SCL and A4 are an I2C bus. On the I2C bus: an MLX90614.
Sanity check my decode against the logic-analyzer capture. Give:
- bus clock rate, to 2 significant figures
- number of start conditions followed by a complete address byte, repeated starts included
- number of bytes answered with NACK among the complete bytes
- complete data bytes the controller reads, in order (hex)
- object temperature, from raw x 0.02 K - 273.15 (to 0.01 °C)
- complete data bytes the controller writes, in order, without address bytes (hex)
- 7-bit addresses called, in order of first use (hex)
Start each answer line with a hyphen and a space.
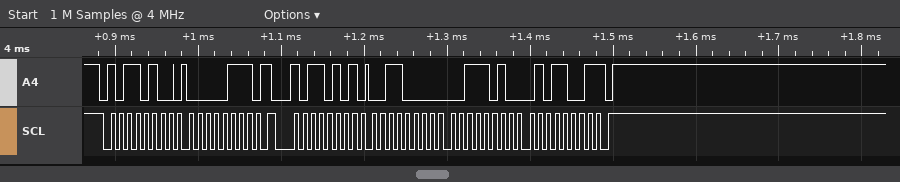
- 100 kHz
- 2
- 1
- 30 3A 59
- 24.77 °C
- 07
- 0x5A
